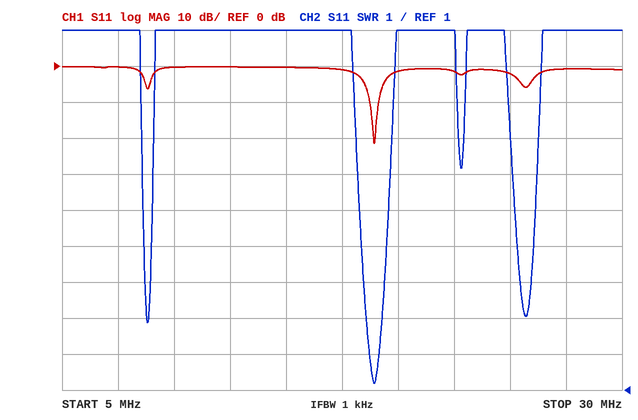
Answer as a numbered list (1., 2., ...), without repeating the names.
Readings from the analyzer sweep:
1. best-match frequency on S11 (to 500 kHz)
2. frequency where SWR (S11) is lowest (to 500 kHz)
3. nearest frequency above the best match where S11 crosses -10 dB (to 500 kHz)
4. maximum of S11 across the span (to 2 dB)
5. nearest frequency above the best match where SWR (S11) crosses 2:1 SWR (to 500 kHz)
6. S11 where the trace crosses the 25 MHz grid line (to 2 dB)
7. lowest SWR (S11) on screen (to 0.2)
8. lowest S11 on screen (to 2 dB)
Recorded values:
1. 19.0 MHz
2. 19.0 MHz
3. 19.0 MHz
4. 0 dB
5. 19.0 MHz
6. -2 dB
7. 1.2
8. -22 dB
